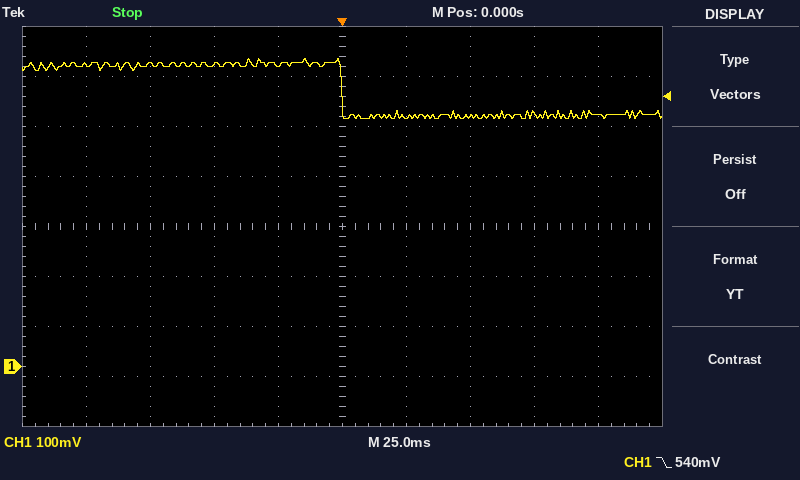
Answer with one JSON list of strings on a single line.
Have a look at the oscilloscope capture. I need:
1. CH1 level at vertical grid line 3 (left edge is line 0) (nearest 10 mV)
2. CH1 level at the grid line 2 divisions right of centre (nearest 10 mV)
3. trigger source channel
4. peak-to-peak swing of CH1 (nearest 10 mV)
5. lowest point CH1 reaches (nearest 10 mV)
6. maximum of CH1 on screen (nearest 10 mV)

["600 mV", "500 mV", "CH1", "120 mV", "500 mV", "620 mV"]
